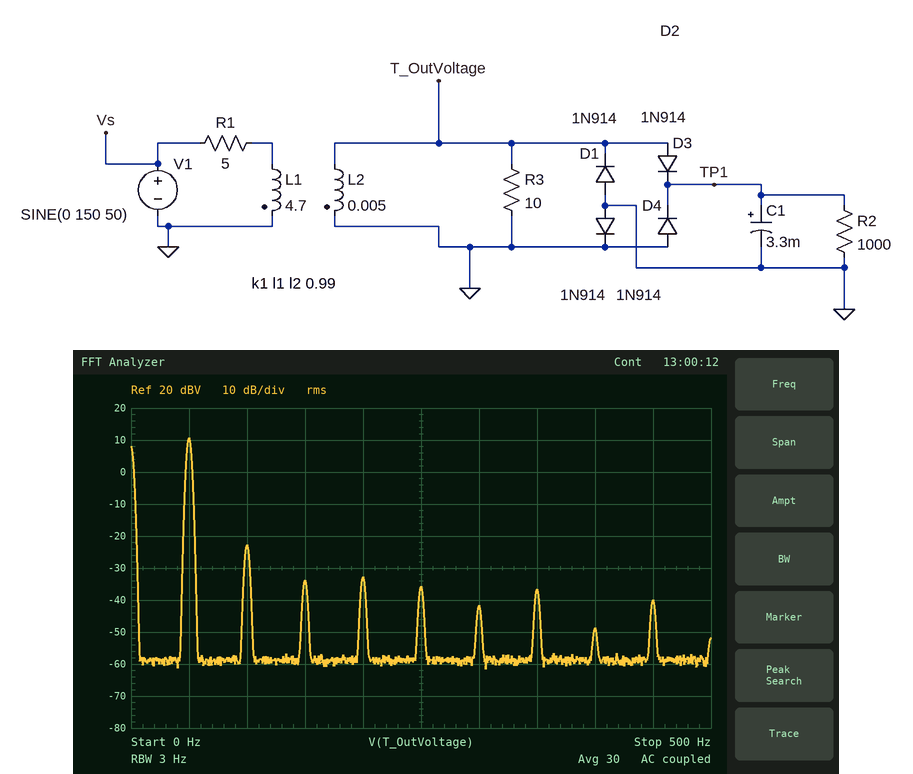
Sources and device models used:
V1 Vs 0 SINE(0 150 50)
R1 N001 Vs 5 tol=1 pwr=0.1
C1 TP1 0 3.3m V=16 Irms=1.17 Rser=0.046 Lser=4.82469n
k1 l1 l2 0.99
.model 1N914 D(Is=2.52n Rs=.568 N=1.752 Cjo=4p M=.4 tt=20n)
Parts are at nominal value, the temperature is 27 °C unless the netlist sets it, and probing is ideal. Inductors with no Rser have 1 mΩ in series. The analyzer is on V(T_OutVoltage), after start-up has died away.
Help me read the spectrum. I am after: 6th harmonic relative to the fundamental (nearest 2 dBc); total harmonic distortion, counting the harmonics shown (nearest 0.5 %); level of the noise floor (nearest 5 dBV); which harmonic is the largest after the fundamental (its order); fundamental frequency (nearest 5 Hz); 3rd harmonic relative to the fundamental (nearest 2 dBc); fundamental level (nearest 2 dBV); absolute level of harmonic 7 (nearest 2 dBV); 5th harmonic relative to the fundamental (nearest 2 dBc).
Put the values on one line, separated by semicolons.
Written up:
-52 dBc; 2.5 %; -60 dBV; 2; 50 Hz; -44 dBc; 10 dBV; -36 dBV; -46 dBc
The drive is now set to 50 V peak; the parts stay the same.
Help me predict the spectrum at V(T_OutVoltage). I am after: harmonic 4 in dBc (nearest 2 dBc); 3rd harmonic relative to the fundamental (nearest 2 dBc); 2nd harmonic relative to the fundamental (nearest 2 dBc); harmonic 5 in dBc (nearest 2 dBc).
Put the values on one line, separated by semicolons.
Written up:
-52 dBc; -40 dBc; -38 dBc; -52 dBc
